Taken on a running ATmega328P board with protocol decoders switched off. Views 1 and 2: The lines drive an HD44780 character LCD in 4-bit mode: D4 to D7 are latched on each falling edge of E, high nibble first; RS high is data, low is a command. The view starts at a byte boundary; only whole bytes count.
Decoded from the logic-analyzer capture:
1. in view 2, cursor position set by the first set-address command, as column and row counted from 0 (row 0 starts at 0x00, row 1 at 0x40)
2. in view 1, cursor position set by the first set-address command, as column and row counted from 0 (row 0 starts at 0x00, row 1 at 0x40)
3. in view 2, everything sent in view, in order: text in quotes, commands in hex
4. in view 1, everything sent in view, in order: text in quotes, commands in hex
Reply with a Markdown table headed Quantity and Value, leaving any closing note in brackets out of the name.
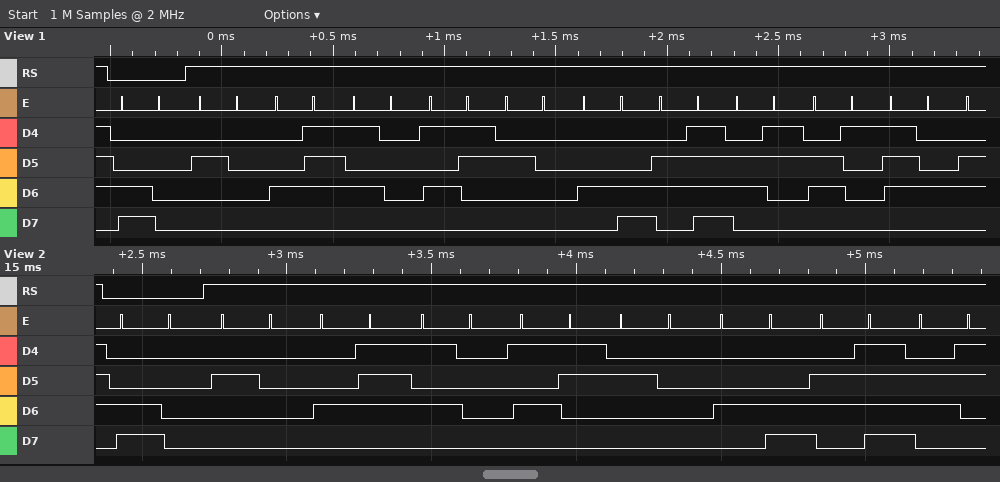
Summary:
| Quantity | Value |
|---|---|
| in view 2, cursor position set by the first set-address command, as column and row counted from 0 | column 0, row 1 |
| in view 1, cursor position set by the first set-address command, as column and row counted from 0 | column 0, row 1 |
| in view 2, everything sent in view, in order: text in quotes, commands in hex | 0xC0 " GPS Loc" |
| in view 1, everything sent in view, in order: text in quotes, commands in hex | 0xC0 " GPS Locat" |
